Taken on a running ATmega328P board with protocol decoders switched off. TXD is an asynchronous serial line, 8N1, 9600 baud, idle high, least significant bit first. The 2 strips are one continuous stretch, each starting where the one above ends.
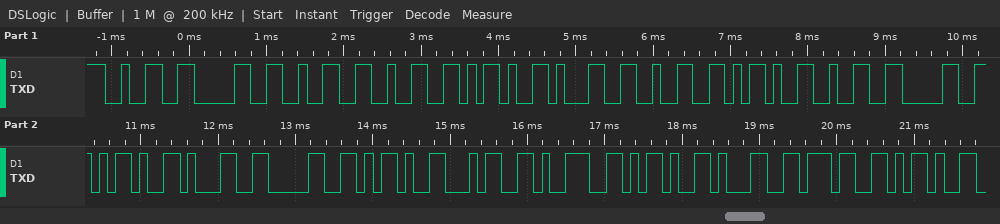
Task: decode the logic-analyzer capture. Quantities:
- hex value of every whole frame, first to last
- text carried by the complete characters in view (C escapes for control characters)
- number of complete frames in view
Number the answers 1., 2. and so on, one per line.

1. 32 30 32 32 2D 31 32 2D 32 30 2D 31 30 2D 34 39 2D 31 37 2D
2. "2022-12-20-10-49-17-"
3. 20
